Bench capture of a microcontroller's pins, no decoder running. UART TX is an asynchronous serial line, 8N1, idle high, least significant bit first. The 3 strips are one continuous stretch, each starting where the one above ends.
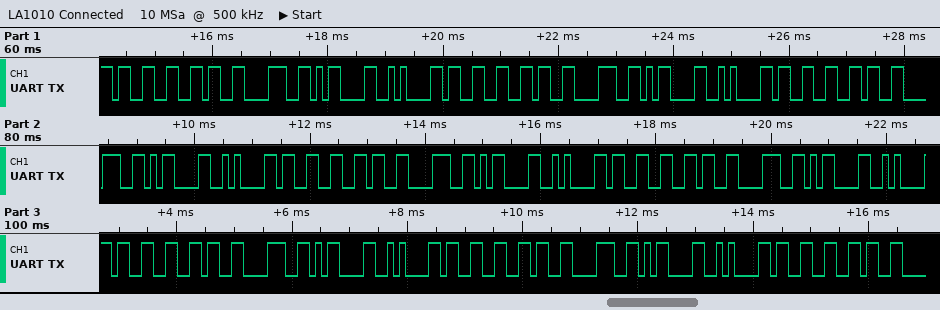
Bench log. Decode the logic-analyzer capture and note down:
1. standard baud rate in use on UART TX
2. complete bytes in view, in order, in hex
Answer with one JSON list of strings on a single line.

["9600 baud", "33 36 38 0D 0A 33 36 38 0D 0A 33 36 38 0D 0A 33 36 38 0D 0A 33 36 38 0D 0A 33 36 38 0D 0A 33 36 38 0D 0A 33 36"]
